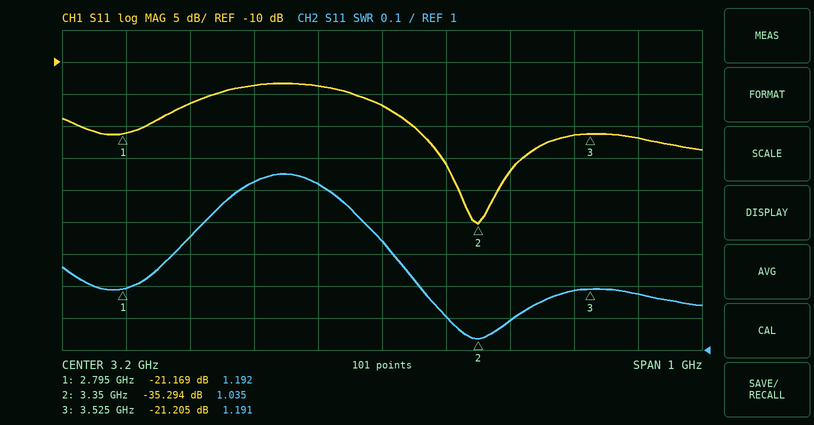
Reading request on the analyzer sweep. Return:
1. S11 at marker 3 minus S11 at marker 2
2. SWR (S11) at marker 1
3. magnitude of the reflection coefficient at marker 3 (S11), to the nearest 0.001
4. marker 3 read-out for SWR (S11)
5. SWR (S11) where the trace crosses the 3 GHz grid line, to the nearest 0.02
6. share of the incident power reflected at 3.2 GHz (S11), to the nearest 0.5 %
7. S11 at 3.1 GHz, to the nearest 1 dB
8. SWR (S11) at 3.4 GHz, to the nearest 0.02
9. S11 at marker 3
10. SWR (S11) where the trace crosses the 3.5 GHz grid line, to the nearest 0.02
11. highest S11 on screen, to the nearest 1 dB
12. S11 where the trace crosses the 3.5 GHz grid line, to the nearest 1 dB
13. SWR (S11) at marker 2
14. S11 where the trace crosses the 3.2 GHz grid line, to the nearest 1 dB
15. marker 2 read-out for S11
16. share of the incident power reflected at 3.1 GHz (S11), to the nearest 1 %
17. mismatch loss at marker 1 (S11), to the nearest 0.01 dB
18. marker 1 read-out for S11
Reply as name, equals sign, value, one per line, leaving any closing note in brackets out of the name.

S11 at marker 3 minus S11 at marker 2 = 14.089 dB
SWR (S11) at marker 1 = 1.192
magnitude of the reflection coefficient at marker 3 (S11), to the nearest 0.001 = 0.087
marker 3 read-out for SWR = 1.191
SWR (S11) where the trace crosses the 3 GHz grid line, to the nearest 0.02 = 1.52
share of the incident power reflected at 3.2 GHz (S11), to the nearest 0.5 % = 2.0 %
S11 at 3.1 GHz, to the nearest 1 dB = -14 dB
SWR (S11) at 3.4 GHz, to the nearest 0.02 = 1.10
S11 at marker 3 = -21.205 dB
SWR (S11) where the trace crosses the 3.5 GHz grid line, to the nearest 0.02 = 1.18
highest S11 on screen, to the nearest 1 dB = -13 dB
S11 where the trace crosses the 3.5 GHz grid line, to the nearest 1 dB = -21 dB
SWR (S11) at marker 2 = 1.035
S11 where the trace crosses the 3.2 GHz grid line, to the nearest 1 dB = -17 dB
marker 2 read-out for S11 = -35.294 dB
share of the incident power reflected at 3.1 GHz (S11), to the nearest 1 % = 4 %
mismatch loss at marker 1 (S11), to the nearest 0.01 dB = 0.03 dB
marker 1 read-out for S11 = -21.169 dB
